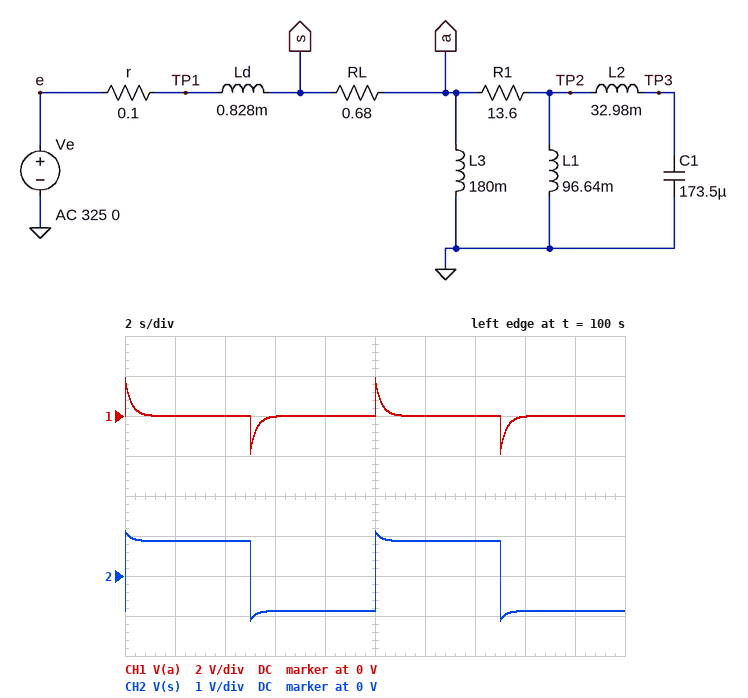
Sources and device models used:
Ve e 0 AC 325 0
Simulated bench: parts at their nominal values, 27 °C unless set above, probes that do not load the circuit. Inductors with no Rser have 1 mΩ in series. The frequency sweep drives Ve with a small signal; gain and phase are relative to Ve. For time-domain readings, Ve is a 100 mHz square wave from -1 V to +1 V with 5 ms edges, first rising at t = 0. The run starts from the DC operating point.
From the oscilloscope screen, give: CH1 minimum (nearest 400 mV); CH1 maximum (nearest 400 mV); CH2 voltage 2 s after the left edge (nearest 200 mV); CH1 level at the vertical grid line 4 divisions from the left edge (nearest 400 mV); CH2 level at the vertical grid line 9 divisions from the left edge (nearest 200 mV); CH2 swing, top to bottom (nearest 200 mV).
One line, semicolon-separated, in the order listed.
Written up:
-2.0 V; 2.0 V; 800 mV; 0 V; -800 mV; 2.2 V
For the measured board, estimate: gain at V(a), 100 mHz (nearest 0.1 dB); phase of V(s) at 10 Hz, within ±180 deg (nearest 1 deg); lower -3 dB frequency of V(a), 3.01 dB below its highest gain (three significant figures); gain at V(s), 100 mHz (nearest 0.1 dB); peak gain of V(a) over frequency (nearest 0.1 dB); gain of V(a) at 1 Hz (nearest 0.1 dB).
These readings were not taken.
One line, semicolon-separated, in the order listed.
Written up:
-16.9 dB; 0 deg; 735 mHz; -1.2 dB; 0 dB; -2.1 dB
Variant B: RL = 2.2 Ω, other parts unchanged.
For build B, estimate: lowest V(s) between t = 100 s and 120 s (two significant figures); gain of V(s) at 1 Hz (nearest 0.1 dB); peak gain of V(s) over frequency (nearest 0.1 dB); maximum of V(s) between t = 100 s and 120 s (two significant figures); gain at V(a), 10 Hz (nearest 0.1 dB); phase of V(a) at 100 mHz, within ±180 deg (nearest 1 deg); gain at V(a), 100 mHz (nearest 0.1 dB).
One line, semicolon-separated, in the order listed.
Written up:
-1.0 V; -0.3 dB; 0 dB; 1.0 V; -1.4 dB; 86 deg; -26.2 dB
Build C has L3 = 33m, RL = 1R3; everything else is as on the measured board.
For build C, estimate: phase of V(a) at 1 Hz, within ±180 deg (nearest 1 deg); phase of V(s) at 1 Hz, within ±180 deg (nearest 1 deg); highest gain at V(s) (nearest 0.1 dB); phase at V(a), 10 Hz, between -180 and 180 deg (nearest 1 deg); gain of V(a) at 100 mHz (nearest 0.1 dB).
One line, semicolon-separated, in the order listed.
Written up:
80 deg; 0 deg; -0.2 dB; 33 deg; -36.6 dB
